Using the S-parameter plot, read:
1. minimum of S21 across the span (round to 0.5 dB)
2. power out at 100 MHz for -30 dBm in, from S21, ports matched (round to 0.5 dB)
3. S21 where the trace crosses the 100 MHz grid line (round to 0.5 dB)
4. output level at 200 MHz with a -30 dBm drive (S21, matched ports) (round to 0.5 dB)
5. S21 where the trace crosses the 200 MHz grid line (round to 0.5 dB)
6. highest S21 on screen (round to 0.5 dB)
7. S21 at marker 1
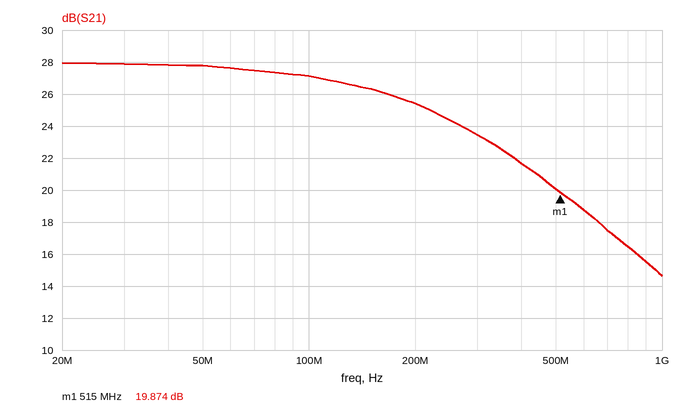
14.5 dB
-3.0 dBm
27.0 dB
-4.5 dBm
25.5 dB
28.0 dB
19.874 dB
